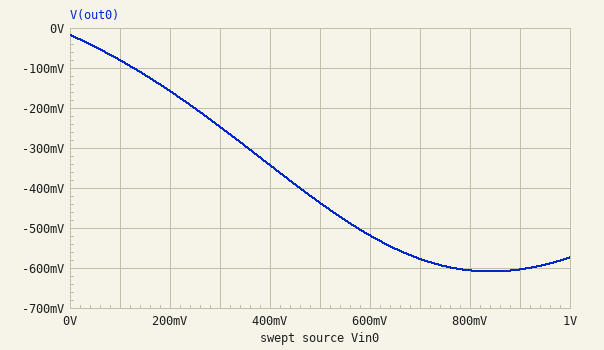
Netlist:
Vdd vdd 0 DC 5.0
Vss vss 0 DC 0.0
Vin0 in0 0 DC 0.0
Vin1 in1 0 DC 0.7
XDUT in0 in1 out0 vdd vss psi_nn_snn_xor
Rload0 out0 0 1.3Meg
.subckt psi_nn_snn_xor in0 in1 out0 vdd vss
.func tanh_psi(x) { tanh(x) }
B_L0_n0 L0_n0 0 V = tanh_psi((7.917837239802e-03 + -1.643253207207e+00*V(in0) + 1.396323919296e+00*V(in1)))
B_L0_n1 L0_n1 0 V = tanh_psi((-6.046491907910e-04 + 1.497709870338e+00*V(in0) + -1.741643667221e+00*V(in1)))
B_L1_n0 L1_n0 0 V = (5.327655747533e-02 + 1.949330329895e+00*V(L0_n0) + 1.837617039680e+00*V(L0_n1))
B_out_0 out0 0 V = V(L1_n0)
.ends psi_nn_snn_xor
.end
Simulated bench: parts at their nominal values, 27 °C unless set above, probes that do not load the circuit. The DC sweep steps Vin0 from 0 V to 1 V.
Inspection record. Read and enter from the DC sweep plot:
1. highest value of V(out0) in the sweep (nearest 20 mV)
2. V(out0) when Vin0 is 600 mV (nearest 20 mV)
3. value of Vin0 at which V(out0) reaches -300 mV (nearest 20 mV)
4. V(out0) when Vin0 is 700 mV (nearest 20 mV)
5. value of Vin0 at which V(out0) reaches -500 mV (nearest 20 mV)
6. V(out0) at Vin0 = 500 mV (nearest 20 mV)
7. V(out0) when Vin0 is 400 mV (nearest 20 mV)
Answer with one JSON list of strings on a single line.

["-20 mV", "-520 mV", "360 mV", "-580 mV", "580 mV", "-440 mV", "-340 mV"]
